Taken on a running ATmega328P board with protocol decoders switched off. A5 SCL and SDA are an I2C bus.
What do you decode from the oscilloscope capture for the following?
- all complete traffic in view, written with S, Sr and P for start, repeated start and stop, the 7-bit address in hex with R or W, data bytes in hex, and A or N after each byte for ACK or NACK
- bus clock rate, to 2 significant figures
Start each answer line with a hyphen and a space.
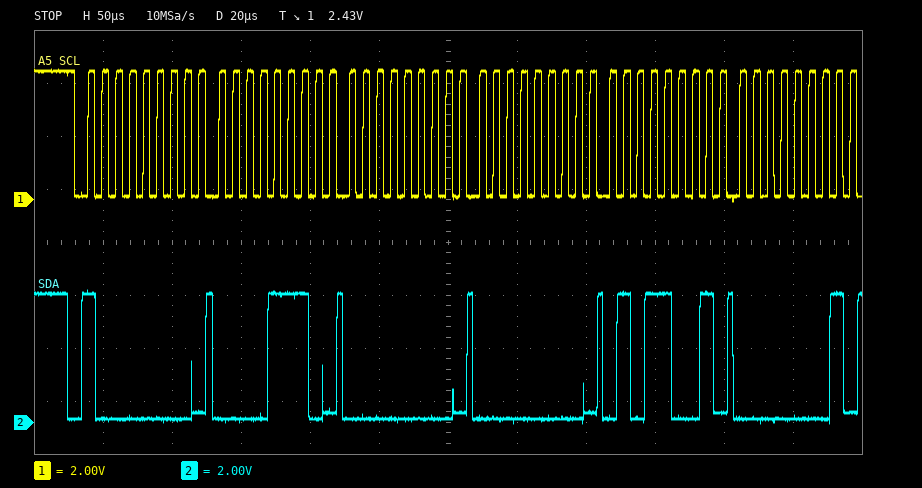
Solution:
- S 40W A 0E A 00 A 00 A 59 A 01 A
- 100 kHz
